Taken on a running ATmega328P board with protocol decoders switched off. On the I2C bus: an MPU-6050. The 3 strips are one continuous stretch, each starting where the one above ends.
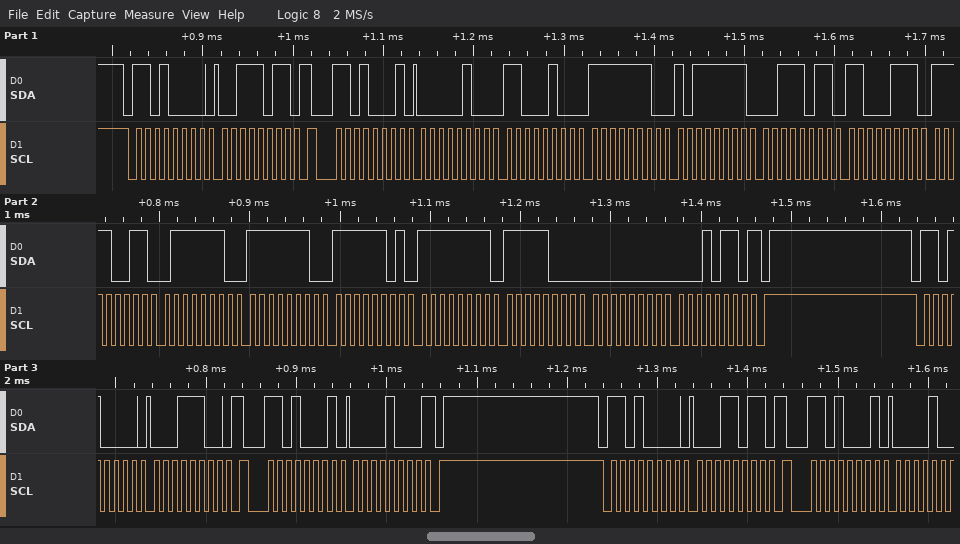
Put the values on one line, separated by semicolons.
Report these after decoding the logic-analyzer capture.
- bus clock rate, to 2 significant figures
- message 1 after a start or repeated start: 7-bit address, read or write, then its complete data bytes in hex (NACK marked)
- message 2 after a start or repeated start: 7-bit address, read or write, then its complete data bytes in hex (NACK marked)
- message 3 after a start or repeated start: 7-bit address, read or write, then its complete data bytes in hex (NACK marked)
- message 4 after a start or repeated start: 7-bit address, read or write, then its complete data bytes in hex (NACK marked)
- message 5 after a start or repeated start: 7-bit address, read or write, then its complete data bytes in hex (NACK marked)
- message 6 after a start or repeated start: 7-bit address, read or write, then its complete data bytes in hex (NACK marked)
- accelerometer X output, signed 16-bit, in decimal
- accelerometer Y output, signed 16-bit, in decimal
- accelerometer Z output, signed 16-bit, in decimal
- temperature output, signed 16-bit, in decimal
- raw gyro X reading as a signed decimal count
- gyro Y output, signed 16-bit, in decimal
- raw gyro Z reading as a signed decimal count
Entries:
100 kHz; 0x68 write: 3B; 0x68 read: 04 C4 FE BF 3B C7 F3 7E FE FD FF F8 00 16 NACK; 0x68 write: 1C; 0x68 read: 08 NACK; 0x68 write: 1B; 0x68 read; 1220; -321; 15303; -3202; -259; -8; 22
